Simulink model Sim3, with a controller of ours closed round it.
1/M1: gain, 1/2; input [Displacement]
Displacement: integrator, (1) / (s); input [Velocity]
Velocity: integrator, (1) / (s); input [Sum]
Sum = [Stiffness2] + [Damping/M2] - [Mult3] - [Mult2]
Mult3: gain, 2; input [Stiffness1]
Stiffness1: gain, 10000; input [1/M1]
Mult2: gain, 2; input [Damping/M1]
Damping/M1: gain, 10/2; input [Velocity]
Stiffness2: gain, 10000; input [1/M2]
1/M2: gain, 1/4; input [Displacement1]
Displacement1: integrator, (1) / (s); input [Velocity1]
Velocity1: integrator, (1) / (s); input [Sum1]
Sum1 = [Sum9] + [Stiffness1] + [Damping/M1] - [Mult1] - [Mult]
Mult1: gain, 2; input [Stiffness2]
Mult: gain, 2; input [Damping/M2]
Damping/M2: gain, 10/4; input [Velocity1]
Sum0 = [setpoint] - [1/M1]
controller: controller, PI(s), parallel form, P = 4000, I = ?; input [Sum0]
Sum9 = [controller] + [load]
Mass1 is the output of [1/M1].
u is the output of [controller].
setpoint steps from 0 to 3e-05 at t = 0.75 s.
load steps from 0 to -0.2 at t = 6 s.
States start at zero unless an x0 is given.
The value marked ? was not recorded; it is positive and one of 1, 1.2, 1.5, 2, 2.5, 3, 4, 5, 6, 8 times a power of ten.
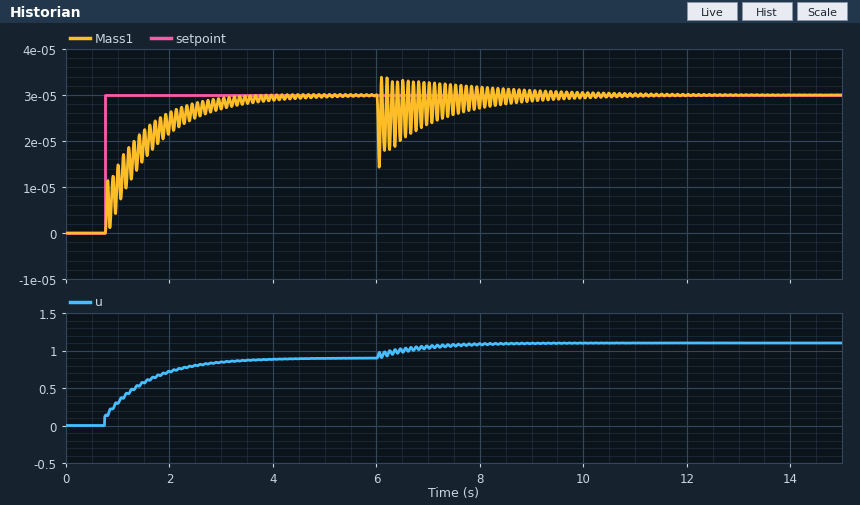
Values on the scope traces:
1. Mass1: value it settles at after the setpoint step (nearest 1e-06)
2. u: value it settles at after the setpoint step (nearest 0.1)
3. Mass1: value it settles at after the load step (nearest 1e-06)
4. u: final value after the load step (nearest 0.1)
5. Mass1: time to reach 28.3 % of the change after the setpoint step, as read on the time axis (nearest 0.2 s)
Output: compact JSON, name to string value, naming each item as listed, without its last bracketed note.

{"Mass1: value it settles at after the setpoint step": "0.000030", "u: value it settles at after the setpoint step": "0.9", "Mass1: value it settles at after the load step": "0.000030", "u: final value after the load step": "1.1", "Mass1: time to reach 28.3 % of the change after the setpoint step, as read on the time axis": "0.8 s"}
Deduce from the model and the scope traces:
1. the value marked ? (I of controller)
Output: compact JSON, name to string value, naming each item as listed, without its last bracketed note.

{"the value marked ?": "40000"}
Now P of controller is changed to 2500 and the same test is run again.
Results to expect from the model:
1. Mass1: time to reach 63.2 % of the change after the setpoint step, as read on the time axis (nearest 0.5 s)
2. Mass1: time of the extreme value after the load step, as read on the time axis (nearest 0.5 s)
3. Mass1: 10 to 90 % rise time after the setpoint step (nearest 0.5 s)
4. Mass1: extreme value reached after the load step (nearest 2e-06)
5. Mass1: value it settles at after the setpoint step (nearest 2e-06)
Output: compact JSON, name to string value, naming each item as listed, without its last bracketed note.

{"Mass1: time to reach 63.2 % of the change after the setpoint step, as read on the time axis": "1.5 s", "Mass1: time of the extreme value after the load step, as read on the time axis": "6.0 s", "Mass1: 10 to 90 % rise time after the setpoint step": "1.5 s", "Mass1: extreme value reached after the load step": "0.000014", "Mass1: value it settles at after the setpoint step": "0.000030"}
